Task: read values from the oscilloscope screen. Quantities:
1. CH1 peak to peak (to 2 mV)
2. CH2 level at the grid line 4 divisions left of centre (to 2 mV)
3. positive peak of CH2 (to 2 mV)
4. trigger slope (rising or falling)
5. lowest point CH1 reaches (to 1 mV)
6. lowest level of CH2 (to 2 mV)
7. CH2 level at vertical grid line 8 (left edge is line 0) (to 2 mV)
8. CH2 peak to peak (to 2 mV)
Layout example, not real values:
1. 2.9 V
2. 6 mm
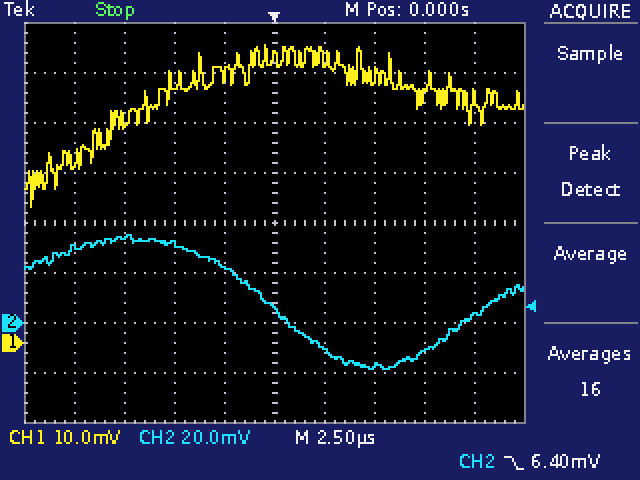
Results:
1. 32 mV
2. 30 mV
3. 36 mV
4. falling
5. 27 mV
6. -18 mV
7. -12 mV
8. 54 mV
